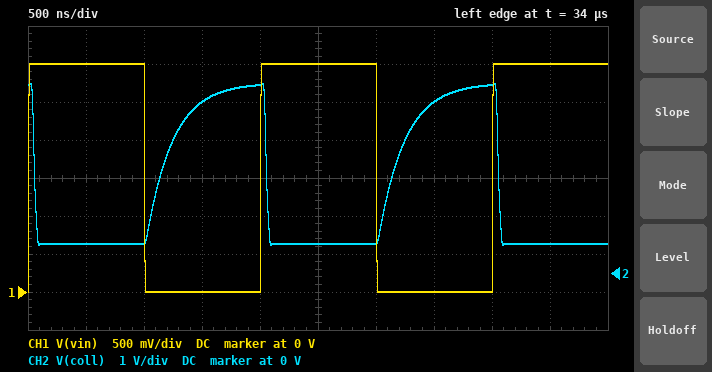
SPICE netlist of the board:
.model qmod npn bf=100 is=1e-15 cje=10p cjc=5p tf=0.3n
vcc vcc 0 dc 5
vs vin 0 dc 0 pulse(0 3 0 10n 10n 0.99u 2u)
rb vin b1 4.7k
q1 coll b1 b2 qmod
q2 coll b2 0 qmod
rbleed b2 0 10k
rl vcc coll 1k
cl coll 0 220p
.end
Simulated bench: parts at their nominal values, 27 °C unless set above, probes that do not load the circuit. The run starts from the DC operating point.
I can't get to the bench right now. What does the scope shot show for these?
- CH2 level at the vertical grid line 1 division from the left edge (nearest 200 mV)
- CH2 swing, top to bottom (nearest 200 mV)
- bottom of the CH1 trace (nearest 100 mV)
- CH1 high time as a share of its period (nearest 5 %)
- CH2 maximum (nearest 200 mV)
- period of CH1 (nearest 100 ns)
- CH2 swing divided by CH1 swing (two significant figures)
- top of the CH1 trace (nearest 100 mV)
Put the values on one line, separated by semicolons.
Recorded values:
800 mV; 4.2 V; 0 V; 50 %; 5.0 V; 2.0 µs; 1.4; 3.0 V
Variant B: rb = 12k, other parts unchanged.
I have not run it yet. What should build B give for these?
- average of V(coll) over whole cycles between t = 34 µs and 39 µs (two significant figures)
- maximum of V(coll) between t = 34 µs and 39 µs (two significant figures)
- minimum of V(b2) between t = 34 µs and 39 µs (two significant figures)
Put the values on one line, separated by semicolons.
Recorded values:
2.6 V; 5.0 V; 9.1 mV
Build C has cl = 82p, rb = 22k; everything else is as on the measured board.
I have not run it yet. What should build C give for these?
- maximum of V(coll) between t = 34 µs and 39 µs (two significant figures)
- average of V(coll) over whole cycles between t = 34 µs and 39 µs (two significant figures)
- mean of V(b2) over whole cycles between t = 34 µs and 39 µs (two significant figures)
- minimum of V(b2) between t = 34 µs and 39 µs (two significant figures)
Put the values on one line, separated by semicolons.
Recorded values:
5.0 V; 2.9 V; 470 mV; -39 mV
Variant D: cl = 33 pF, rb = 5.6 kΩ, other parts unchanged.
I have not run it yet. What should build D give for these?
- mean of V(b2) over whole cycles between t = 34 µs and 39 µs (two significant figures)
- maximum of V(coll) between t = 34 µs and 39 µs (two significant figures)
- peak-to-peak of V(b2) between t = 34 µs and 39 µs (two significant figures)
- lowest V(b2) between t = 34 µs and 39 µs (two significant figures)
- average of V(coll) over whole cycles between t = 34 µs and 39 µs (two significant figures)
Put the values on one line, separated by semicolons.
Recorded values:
460 mV; 5.1 V; 750 mV; 9.4 mV; 2.8 V
